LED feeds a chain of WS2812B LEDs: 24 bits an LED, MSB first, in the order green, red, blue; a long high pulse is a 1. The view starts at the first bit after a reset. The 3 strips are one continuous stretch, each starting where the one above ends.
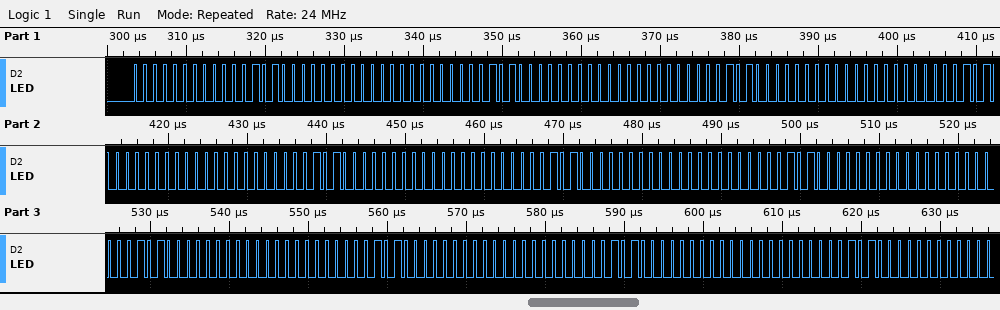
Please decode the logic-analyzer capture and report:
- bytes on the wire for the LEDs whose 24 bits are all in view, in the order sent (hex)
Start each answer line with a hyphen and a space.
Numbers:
- 00 0A 00 00 0A 00 00 0A 00 00 0A 00 00 0A 00 00 0A 00 00 0A 00 00 0A 00 00 0A 00 00 0A 00 00 0A 00
